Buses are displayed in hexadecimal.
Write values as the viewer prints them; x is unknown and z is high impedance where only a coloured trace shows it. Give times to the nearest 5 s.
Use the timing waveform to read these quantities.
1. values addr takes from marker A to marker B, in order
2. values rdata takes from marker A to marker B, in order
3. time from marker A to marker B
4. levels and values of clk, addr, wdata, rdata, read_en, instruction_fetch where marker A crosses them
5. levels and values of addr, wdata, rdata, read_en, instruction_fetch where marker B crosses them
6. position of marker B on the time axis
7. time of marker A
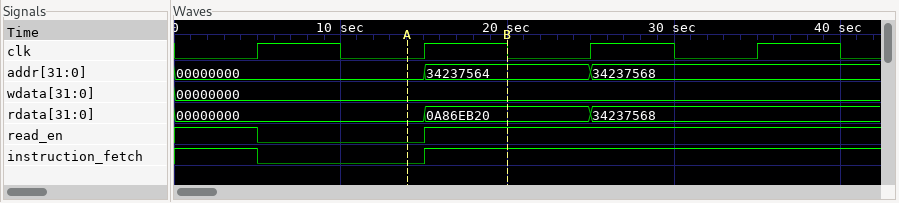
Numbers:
00000000, 34237564
00000000, 0A86EB20
5 s
clk=0, addr=00000000, wdata=00000000, rdata=00000000, read_en=0, instruction_fetch=0
addr=34237564, wdata=00000000, rdata=0A86EB20, read_en=1, instruction_fetch=1
20 s
15 s
